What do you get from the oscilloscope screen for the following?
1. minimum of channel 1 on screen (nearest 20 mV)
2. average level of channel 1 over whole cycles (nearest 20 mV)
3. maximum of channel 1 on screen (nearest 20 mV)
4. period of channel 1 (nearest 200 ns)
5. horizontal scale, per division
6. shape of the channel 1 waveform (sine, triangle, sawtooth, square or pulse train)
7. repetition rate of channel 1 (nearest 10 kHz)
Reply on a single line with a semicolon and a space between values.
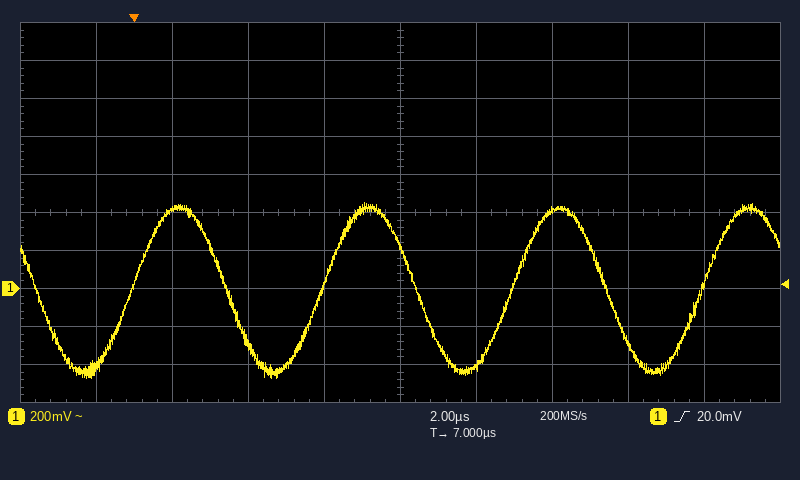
-480 mV; 0 mV; 460 mV; 5.0 µs; 2 µs; sine; 200 kHz
